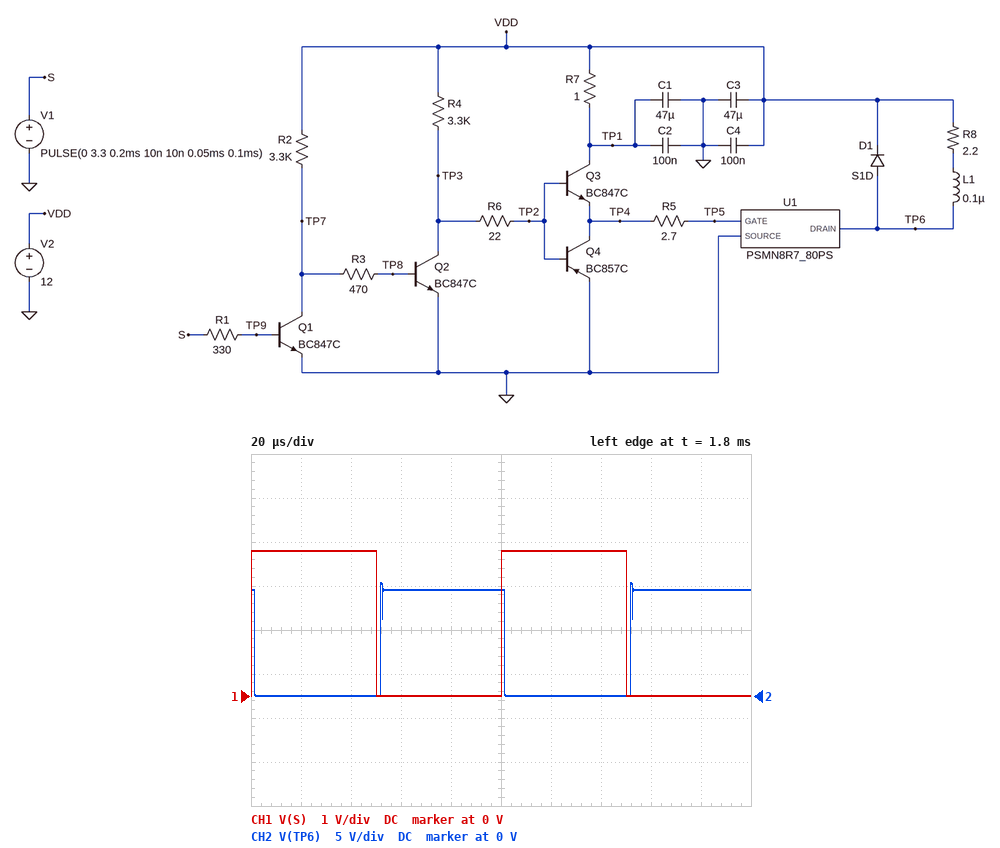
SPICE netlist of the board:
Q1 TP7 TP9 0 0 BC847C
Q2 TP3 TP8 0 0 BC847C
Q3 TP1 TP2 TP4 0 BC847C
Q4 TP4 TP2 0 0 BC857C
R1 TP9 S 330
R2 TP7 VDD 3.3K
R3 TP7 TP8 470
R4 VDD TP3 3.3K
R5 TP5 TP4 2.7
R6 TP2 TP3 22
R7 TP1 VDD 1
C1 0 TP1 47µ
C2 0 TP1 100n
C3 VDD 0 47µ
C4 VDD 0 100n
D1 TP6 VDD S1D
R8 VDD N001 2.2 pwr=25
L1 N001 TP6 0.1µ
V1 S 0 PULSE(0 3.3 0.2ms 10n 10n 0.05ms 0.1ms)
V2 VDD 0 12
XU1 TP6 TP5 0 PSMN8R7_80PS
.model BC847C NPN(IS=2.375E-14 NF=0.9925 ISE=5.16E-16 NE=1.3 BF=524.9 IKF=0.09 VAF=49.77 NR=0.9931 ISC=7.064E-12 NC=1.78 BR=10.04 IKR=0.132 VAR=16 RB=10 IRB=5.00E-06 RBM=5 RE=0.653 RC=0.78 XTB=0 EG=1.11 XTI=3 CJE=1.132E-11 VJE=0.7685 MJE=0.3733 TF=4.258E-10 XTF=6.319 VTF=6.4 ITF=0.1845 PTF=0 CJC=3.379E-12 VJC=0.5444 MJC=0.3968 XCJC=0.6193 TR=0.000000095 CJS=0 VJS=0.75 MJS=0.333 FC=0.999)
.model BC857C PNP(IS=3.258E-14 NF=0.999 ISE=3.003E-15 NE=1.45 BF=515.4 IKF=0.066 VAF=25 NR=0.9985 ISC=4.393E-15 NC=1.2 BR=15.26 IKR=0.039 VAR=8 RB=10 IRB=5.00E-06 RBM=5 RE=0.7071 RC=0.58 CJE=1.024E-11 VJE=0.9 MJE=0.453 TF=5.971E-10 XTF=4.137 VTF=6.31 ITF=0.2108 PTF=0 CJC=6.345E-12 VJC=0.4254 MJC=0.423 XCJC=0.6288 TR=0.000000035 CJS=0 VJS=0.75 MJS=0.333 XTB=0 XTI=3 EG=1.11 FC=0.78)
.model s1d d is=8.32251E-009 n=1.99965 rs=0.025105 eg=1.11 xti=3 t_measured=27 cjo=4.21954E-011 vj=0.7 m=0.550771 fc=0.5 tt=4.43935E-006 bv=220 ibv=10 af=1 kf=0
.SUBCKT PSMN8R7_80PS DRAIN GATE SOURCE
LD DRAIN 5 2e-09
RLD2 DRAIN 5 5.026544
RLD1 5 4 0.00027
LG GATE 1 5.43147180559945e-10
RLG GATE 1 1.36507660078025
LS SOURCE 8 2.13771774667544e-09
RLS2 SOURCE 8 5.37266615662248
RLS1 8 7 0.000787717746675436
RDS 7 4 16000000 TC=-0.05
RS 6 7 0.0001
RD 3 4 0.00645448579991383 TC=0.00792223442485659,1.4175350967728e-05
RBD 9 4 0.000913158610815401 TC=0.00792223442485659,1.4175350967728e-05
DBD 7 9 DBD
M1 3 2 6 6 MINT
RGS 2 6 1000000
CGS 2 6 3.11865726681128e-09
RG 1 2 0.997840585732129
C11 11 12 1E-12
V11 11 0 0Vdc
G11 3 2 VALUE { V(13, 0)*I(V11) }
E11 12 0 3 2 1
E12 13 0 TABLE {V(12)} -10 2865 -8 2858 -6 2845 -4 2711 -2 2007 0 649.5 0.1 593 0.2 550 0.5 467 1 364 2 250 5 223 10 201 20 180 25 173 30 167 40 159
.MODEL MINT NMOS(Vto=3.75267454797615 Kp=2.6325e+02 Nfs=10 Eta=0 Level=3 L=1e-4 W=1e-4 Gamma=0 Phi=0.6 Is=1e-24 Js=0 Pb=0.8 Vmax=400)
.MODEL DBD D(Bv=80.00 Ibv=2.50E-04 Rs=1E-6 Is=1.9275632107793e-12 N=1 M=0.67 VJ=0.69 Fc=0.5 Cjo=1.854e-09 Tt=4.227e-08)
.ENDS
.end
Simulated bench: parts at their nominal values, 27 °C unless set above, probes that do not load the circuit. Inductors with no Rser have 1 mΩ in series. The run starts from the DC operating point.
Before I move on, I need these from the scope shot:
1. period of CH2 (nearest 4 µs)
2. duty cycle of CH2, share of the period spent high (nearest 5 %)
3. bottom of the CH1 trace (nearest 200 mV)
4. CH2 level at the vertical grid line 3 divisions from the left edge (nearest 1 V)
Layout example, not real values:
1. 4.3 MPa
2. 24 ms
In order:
1. 100 µs
2. 50 %
3. 0 V
4. 12 V
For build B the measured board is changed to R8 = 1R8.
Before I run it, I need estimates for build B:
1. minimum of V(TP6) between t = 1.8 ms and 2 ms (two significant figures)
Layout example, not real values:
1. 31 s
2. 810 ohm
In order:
1. 52 mV
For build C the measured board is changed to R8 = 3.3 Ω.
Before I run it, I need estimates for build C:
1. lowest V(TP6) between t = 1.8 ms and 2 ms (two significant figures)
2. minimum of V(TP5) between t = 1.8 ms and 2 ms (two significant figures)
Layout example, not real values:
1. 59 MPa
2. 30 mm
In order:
1. 22 mV
2. -190 mV
